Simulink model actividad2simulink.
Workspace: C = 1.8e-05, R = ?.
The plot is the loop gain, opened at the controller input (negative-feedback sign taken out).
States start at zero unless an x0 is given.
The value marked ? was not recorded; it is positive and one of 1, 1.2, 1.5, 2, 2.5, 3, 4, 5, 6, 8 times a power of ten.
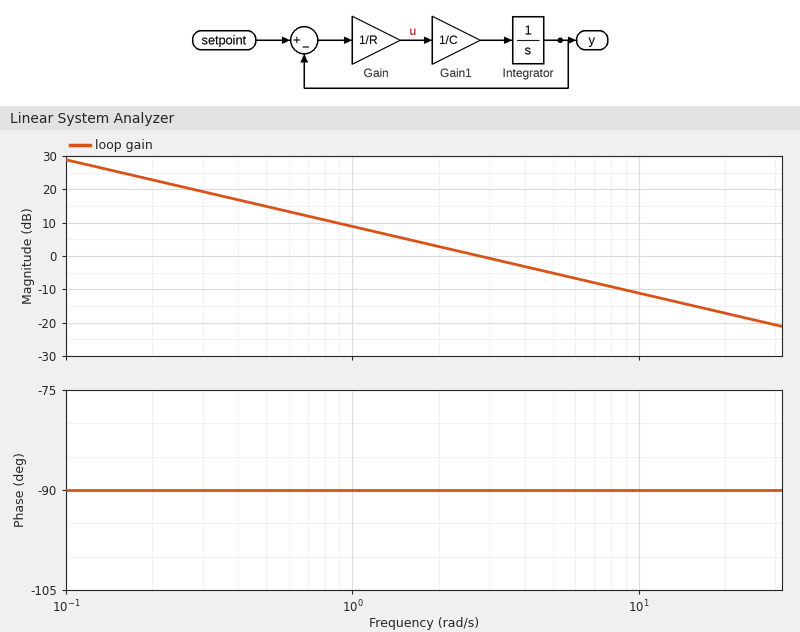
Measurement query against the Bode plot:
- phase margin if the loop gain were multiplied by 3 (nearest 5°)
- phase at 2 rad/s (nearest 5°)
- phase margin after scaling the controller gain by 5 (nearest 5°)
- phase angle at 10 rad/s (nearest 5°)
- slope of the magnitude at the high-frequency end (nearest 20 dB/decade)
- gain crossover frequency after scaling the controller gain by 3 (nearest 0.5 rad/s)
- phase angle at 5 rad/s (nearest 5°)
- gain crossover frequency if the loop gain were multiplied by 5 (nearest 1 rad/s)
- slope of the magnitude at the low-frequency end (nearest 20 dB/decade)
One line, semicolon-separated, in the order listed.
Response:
90°; -90°; 90°; -90°; -20 dB/decade; 8.5 rad/s; -90°; 14 rad/s; -20 dB/decade
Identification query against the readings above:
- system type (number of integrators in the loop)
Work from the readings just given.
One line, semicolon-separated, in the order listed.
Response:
1
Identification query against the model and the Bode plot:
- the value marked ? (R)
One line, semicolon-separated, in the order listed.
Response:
20000
